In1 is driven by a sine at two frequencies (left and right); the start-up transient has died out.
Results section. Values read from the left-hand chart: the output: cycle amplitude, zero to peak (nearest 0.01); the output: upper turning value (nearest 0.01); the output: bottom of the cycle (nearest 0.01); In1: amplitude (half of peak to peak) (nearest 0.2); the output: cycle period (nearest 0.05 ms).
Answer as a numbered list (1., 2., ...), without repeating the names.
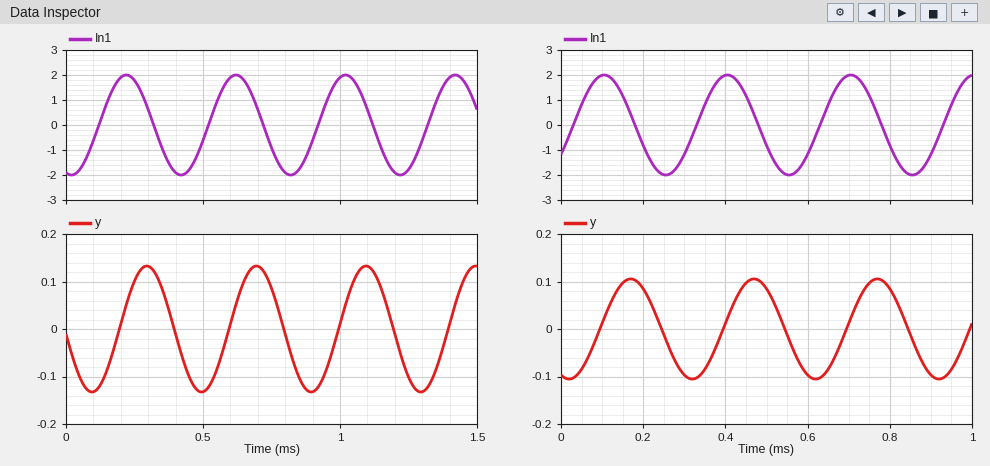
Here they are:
1. 0.13
2. 0.13
3. -0.13
4. 2.0
5. 0.40 ms
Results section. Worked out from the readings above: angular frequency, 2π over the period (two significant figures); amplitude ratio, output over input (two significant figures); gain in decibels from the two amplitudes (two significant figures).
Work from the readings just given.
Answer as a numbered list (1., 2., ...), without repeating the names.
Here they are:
1. 16 rad/ms
2. 0.065
3. -24 dB
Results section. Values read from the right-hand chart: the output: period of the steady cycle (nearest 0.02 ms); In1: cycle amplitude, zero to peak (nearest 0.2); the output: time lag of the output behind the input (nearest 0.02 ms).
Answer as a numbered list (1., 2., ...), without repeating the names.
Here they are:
1. 0.30 ms
2. 2.0
3. 0.06 ms
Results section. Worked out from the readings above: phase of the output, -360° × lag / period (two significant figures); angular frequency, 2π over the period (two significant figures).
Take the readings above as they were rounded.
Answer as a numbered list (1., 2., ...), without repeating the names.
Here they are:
1. -72°
2. 21 rad/ms
